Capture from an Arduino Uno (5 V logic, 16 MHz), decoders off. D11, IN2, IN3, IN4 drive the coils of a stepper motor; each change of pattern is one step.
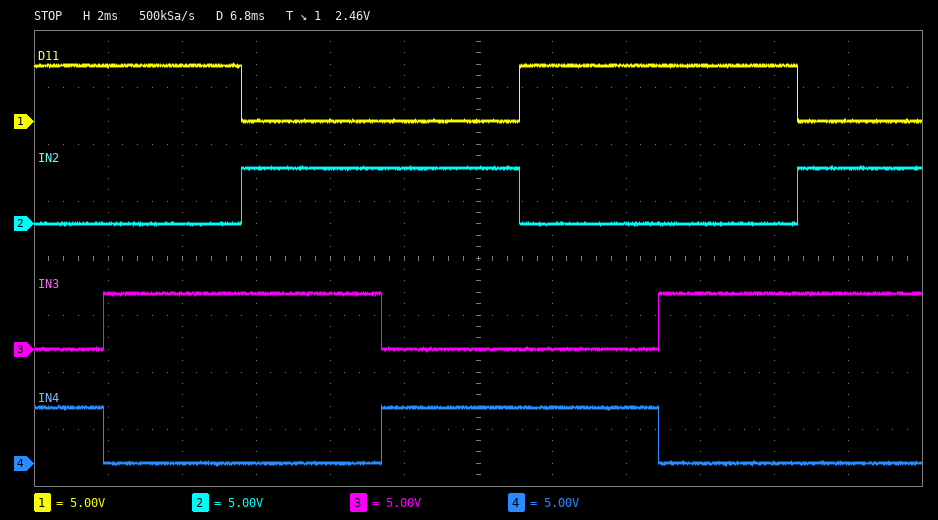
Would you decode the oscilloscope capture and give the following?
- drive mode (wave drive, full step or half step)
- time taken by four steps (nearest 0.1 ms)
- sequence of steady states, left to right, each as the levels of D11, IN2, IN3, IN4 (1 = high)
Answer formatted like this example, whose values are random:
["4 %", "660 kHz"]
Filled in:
["full step", "15.0 ms", "1001 1010 0110 0101 1001 1010 0110"]
